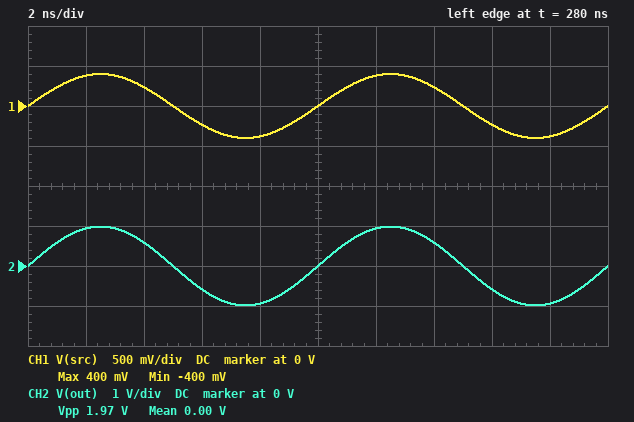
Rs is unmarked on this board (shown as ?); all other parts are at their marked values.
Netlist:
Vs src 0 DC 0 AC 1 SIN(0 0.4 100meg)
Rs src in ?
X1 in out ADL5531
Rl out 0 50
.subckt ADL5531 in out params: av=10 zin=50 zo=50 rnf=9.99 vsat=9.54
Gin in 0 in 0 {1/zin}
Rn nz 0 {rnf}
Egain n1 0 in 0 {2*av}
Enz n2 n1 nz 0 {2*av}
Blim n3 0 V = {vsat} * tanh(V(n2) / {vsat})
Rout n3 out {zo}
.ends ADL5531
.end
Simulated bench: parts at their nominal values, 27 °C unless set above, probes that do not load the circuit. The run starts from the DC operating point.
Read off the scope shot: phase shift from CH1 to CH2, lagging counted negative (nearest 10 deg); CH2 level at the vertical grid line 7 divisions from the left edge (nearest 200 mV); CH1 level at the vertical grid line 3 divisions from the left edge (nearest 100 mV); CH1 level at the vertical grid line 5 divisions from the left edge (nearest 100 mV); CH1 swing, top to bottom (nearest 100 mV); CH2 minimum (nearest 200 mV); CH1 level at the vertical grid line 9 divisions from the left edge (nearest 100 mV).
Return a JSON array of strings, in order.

["0 deg", "600 mV", "-200 mV", "0 V", "800 mV", "-1.0 V", "-400 mV"]
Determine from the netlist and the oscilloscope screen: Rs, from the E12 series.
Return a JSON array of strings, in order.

["150 Ω"]
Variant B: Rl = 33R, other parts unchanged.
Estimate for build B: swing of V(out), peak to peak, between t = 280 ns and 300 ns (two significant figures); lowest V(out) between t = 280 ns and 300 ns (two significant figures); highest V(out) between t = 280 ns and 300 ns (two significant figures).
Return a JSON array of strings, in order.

["1.6 V", "-780 mV", "780 mV"]
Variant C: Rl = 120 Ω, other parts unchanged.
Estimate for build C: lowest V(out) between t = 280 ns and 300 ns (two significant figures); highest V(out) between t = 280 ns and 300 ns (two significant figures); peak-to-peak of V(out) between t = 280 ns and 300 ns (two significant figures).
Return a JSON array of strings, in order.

["-1.4 V", "1.4 V", "2.8 V"]
